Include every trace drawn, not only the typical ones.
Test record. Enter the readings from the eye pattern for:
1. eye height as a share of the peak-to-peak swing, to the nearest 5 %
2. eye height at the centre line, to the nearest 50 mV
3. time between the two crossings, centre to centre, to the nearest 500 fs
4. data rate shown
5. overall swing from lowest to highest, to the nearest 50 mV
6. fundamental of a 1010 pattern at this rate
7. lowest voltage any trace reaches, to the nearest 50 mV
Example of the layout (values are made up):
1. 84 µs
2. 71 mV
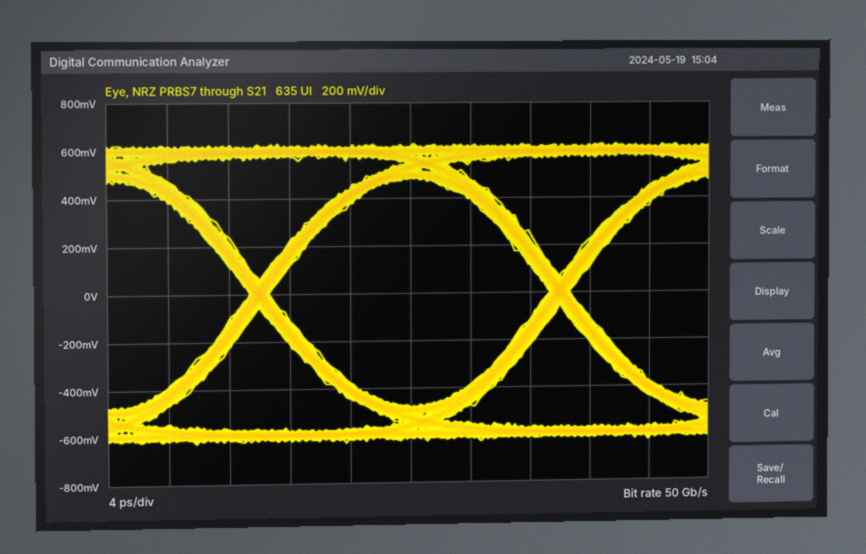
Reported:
1. 75 %
2. 950 mV
3. 20.0 ps
4. 50 Gb/s
5. 1.25 V
6. 25 GHz
7. -650 mV
